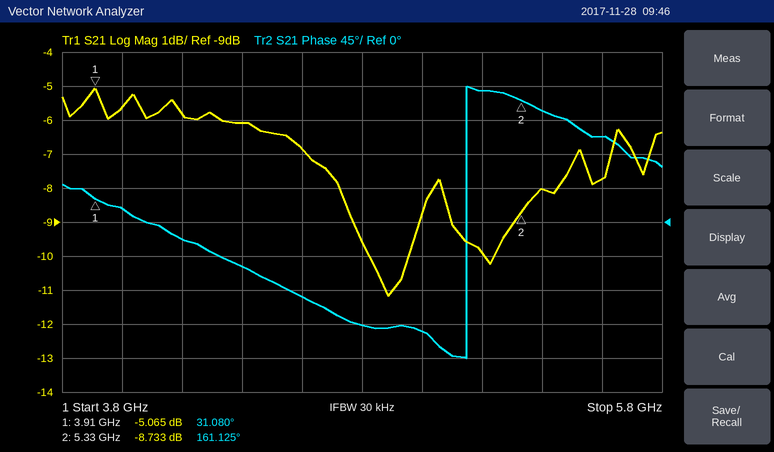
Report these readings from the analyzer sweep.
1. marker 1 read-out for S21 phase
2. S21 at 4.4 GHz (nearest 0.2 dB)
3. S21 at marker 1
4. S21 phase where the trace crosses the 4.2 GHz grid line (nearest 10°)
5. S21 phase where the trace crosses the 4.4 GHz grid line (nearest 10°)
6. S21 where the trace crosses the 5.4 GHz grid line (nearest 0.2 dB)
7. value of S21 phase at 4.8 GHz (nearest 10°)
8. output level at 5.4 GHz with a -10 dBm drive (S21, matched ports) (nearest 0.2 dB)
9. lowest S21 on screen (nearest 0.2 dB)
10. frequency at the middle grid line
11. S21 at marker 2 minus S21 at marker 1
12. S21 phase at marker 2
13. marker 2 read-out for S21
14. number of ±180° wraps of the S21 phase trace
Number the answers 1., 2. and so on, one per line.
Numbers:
1. 31.080°
2. -6.0 dB
3. -5.065 dB
4. -20°
5. -60°
6. -8.0 dB
7. -140°
8. -18.0 dBm
9. -11.2 dB
10. 4.8 GHz
11. -3.668 dB
12. 161.125°
13. -8.733 dB
14. 1
